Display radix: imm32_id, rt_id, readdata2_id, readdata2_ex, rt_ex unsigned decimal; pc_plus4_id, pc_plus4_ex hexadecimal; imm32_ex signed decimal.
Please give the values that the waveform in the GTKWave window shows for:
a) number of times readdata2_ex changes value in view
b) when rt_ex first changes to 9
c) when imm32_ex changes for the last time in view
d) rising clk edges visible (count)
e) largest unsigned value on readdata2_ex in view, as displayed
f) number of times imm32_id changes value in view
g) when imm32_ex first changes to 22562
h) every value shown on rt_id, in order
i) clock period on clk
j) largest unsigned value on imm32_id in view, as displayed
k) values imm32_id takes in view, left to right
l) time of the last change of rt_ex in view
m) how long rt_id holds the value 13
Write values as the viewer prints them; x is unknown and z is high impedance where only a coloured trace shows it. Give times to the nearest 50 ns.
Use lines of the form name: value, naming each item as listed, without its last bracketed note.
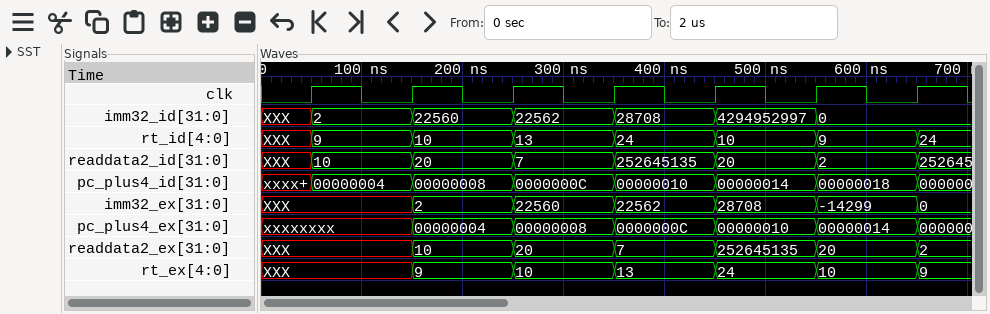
number of times readdata2_ex changes value in view: 6
when rt_ex first changes to 9: 150 ns
when imm32_ex changes for the last time in view: 650 ns
rising clk edges visible: 7
largest unsigned value on readdata2_ex in view, as displayed: 252645135
number of times imm32_id changes value in view: 6
when imm32_ex first changes to 22562: 350 ns
every value shown on rt_id, in order: XXX, 9, 10, 13, 24, 10, 9, 24
clock period on clk: 100 ns
largest unsigned value on imm32_id in view, as displayed: 4294952997
values imm32_id takes in view, left to right: XXX, 2, 22560, 22562, 28708, 4294952997, 0
time of the last change of rt_ex in view: 650 ns
how long rt_id holds the value 13: 100 ns
